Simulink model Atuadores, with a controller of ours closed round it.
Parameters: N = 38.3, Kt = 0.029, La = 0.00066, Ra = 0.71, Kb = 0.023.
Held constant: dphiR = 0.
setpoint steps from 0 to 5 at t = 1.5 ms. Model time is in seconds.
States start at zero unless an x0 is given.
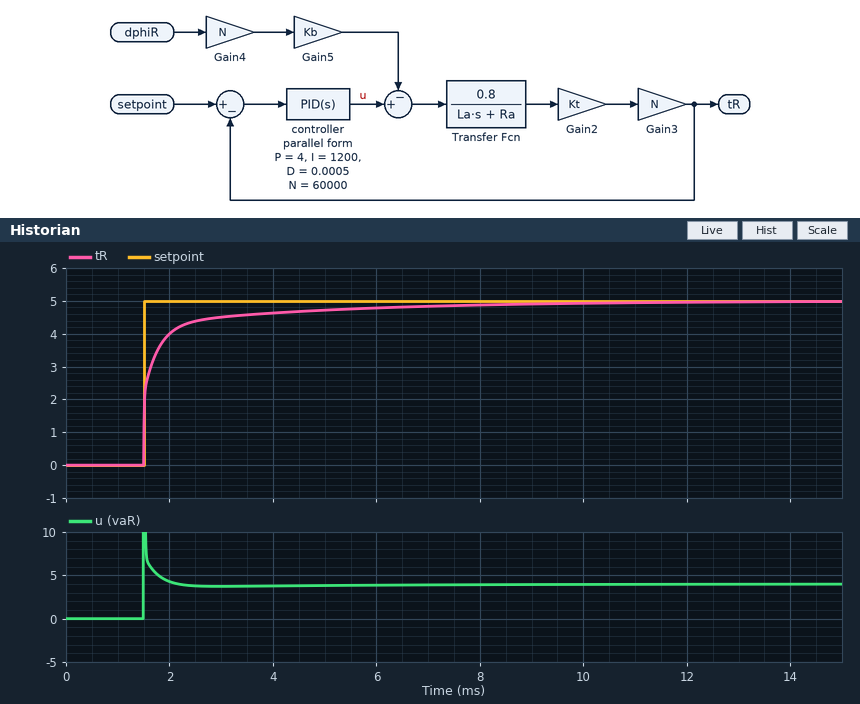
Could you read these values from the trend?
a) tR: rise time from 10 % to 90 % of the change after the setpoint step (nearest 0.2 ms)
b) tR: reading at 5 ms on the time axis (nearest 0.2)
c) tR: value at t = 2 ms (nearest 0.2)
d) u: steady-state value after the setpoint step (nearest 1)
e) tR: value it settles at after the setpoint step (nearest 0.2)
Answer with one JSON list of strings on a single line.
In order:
["1.4 ms", "4.8", "4.0", "4", "5.0"]
